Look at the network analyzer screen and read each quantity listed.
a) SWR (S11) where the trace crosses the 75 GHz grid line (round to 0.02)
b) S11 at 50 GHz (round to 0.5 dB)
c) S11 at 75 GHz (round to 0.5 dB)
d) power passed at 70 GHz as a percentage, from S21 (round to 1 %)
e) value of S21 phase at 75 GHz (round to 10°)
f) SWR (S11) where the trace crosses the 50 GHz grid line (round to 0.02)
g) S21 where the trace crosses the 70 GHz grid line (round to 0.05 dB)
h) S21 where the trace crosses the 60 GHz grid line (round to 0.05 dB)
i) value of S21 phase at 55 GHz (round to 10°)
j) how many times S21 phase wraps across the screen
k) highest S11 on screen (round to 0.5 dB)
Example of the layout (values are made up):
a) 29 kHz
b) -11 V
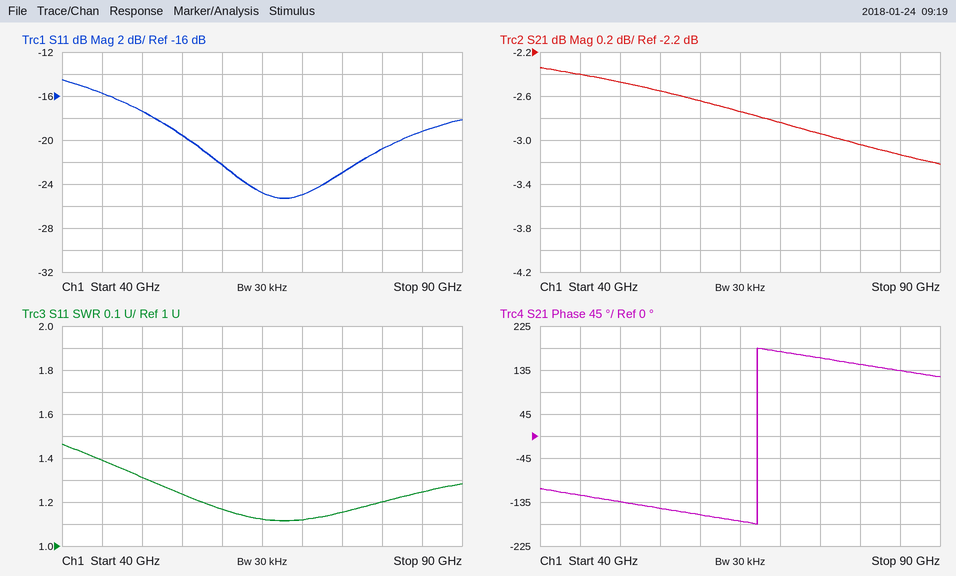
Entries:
a) 1.16
b) -17.5 dB
c) -23.0 dB
d) 52 %
e) 160°
f) 1.32
g) -2.85 dB
h) -2.65 dB
i) -150°
j) 1
k) -14.5 dB
